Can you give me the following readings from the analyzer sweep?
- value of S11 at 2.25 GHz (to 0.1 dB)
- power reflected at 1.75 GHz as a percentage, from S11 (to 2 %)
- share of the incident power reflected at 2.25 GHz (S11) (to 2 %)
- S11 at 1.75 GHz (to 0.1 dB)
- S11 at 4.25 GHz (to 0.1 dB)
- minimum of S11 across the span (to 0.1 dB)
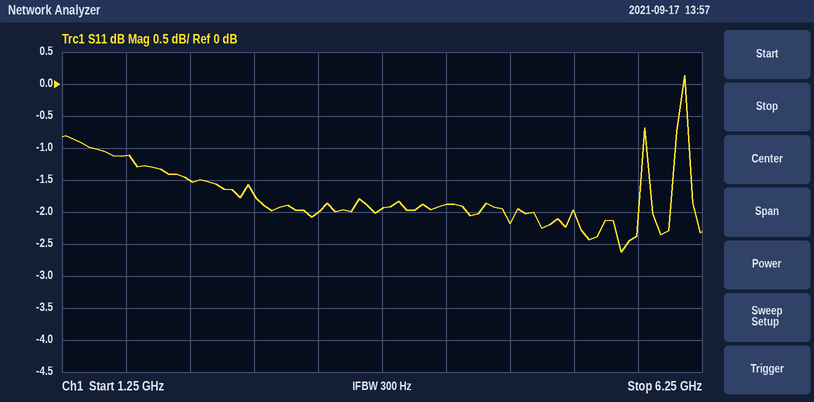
-1.5 dB
78 %
70 %
-1.1 dB
-1.9 dB
-2.6 dB
